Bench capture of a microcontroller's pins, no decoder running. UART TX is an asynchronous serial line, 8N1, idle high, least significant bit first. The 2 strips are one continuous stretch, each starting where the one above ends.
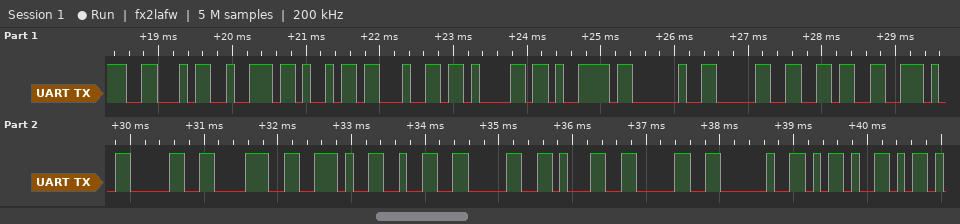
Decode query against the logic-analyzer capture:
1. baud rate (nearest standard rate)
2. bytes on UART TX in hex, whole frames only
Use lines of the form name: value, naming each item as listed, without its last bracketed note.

baud rate: 9600 baud
bytes on UART TX in hex, whole frames only: 0x46 0x72 0x69 0x64 0x61 0x79 0x20 0x30 0x36 0x2E 0x30 0x38 0x2E 0x32 0x30 0x31 0x30 0x20 0x2D
